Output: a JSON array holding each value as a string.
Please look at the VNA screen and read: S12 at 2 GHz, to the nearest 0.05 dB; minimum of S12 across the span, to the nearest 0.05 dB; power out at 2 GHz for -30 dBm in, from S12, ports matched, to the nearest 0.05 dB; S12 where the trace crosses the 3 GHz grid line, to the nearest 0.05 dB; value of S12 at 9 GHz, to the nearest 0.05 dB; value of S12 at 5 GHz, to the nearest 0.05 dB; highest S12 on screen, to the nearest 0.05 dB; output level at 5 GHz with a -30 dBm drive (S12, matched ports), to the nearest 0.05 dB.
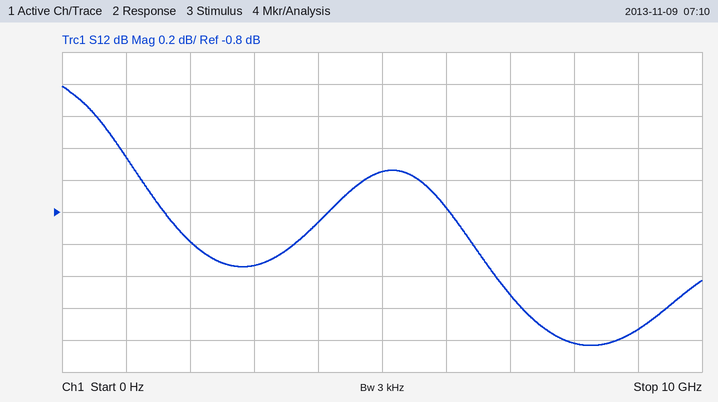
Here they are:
["-1.00 dB", "-1.65 dB", "-31.00 dBm", "-1.15 dB", "-1.55 dB", "-0.55 dB", "0.00 dB", "-30.55 dBm"]
